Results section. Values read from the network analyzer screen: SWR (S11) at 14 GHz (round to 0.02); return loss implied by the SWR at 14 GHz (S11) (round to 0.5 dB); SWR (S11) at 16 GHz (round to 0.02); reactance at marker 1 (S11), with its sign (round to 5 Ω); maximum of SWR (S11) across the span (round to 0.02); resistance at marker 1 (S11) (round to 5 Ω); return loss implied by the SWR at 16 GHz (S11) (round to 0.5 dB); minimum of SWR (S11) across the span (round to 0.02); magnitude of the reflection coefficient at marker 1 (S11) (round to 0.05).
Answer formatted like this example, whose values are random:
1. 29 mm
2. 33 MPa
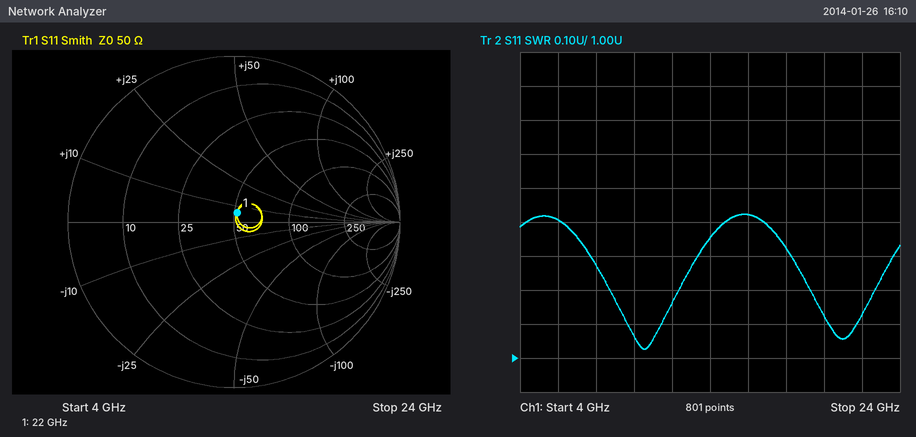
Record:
1. 1.36
2. 16.5 dB
3. 1.42
4. +5 Ω
5. 1.42
6. 50 Ω
7. 15.0 dB
8. 1.02
9. 0.05
